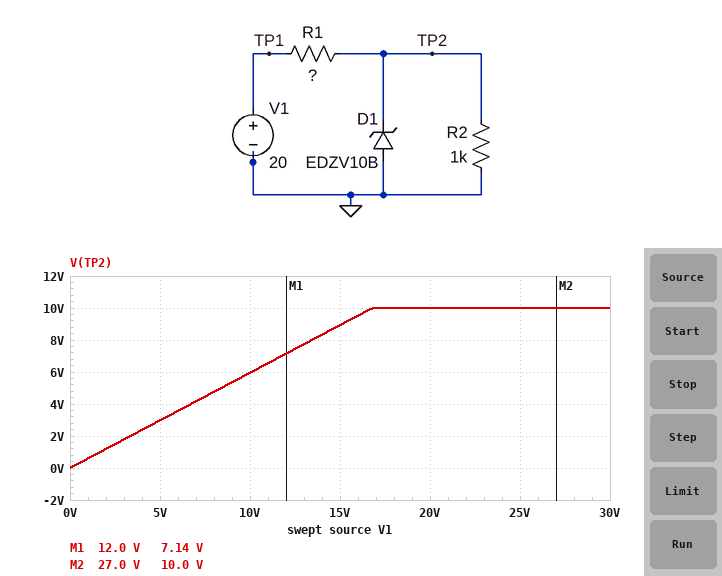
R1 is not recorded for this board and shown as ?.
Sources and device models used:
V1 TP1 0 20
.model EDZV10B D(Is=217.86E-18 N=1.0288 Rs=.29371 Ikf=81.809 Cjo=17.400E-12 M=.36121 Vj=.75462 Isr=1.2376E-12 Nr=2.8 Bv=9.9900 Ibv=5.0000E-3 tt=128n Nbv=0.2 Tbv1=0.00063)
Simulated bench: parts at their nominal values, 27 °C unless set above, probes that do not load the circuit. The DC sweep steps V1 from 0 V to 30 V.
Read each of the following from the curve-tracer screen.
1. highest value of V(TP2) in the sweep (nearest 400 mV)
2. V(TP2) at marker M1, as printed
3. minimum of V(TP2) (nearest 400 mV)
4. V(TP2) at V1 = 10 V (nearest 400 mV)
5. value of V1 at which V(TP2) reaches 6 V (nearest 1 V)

10.0 V
7.14 V
0 V
6.0 V
10 V
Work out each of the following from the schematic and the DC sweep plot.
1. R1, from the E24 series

680 Ω
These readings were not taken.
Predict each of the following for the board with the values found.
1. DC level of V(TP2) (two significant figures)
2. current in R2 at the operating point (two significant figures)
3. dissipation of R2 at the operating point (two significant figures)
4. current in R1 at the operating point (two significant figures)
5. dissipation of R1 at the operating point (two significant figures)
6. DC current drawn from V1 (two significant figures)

10 V
10 mA
100 mW
15 mA
150 mW
15 mA
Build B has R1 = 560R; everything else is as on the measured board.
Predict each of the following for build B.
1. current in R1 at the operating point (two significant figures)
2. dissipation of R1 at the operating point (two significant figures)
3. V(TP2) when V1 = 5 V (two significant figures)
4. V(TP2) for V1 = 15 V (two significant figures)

18 mA
180 mW
3.2 V
9.6 V
